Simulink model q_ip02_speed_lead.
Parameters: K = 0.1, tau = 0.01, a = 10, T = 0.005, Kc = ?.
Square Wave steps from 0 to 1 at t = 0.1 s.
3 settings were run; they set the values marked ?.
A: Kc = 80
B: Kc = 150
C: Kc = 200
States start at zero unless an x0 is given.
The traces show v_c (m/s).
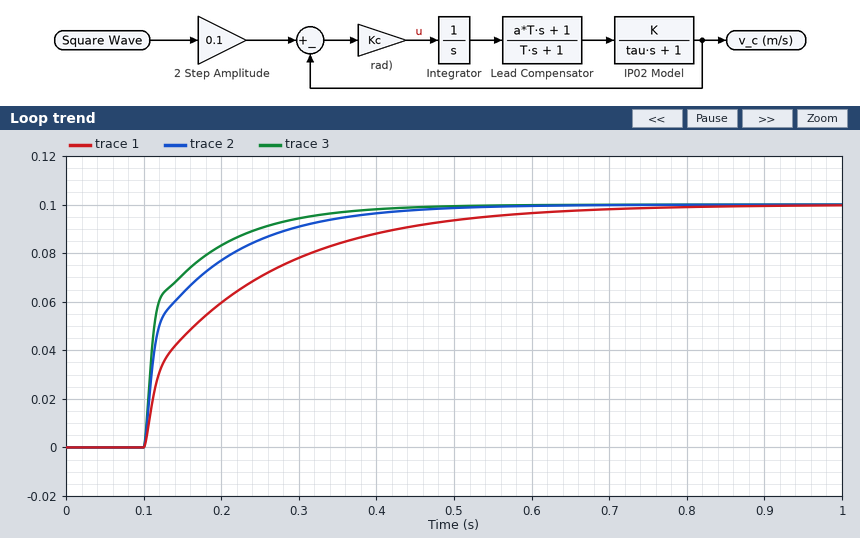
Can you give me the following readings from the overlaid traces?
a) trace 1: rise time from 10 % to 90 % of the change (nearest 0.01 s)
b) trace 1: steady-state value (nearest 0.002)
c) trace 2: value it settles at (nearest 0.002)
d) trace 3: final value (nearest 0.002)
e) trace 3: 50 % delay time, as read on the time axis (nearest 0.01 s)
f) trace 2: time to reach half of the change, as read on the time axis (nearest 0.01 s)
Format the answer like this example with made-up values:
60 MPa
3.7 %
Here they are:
0.32 s
0.100
0.100
0.100
0.11 s
0.12 s
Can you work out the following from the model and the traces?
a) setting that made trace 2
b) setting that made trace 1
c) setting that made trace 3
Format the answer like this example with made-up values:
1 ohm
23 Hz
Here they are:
B
A
C
